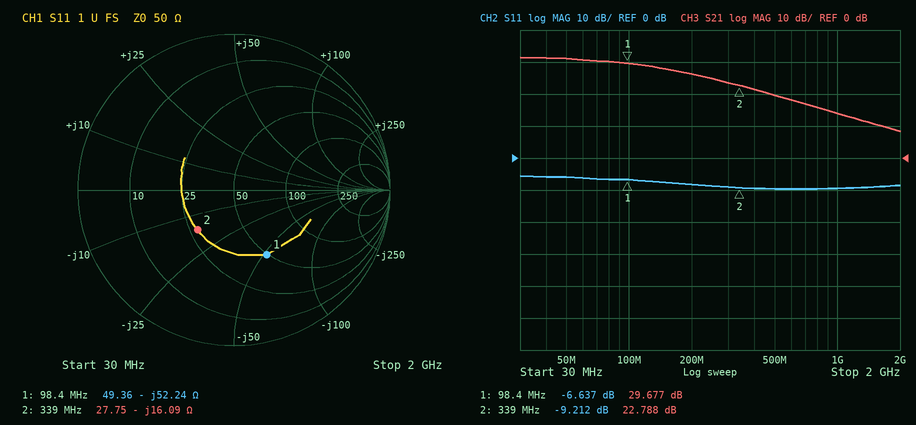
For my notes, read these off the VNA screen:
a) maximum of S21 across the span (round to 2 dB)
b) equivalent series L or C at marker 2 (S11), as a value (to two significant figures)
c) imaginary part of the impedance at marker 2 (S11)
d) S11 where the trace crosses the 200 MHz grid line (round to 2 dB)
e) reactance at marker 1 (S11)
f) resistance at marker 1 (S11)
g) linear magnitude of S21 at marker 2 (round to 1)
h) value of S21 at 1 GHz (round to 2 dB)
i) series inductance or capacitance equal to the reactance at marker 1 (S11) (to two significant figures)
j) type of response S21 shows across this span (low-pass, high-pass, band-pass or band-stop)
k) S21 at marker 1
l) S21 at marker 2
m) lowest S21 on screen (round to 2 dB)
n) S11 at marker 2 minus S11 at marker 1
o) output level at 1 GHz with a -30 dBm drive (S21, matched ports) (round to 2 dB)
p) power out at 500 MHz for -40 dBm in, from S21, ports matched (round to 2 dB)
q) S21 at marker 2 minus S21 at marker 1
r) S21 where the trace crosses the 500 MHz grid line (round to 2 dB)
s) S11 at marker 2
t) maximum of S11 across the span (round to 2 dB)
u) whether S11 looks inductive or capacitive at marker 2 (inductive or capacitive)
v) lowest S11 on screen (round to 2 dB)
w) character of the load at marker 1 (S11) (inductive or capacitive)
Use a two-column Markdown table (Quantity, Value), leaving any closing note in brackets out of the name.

| Quantity | Value |
|---|---|
| maximum of S21 across the span | 32 dB |
| equivalent series L or C at marker 2 (S11), as a value | 29 pF |
| imaginary part of the impedance at marker 2 | -16.09 Ω |
| S11 where the trace crosses the 200 MHz grid line | -8 dB |
| reactance at marker 1 | -52.24 Ω |
| resistance at marker 1 | 49.36 Ω |
| linear magnitude of S21 at marker 2 | 14 |
| value of S21 at 1 GHz | 14 dB |
| series inductance or capacitance equal to the reactance at marker 1 (S11) | 31 pF |
| type of response S21 shows across this span | low-pass |
| S21 at marker 1 | 29.677 dB |
| S21 at marker 2 | 22.788 dB |
| lowest S21 on screen | 8 dB |
| S11 at marker 2 minus S11 at marker 1 | -2.575 dB |
| output level at 1 GHz with a -30 dBm drive (S21, matched ports) | -16 dBm |
| power out at 500 MHz for -40 dBm in, from S21, ports matched | -20 dBm |
| S21 at marker 2 minus S21 at marker 1 | -6.889 dB |
| S21 where the trace crosses the 500 MHz grid line | 20 dB |
| S11 at marker 2 | -9.212 dB |
| maximum of S11 across the span | -6 dB |
| whether S11 looks inductive or capacitive at marker 2 | capacitive |
| lowest S11 on screen | -10 dB |
| character of the load at marker 1 (S11) | capacitive |
